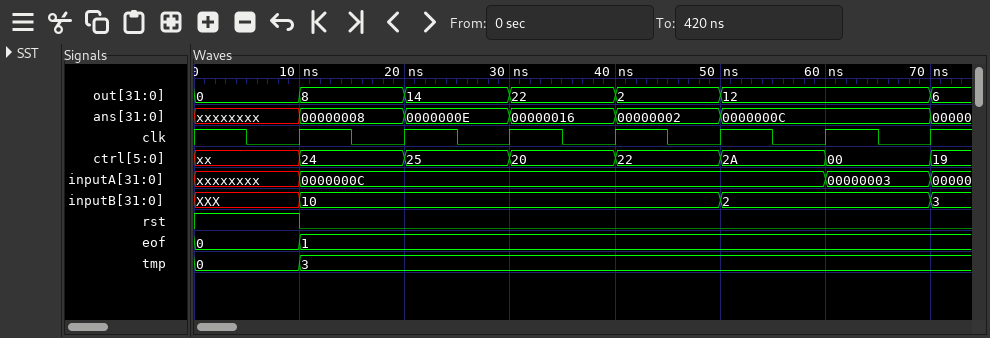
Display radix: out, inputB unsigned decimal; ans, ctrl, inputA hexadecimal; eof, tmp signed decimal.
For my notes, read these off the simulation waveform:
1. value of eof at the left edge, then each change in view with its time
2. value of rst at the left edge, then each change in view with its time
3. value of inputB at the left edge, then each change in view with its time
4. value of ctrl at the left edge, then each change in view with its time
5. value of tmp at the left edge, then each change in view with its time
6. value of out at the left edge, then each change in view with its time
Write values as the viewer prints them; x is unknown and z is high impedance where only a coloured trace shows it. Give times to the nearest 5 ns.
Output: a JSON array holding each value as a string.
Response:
["0, 1 at 10 ns", "1, 0 at 10 ns", "XXX, 10 at 10 ns, 2 at 50 ns, 3 at 70 ns", "xx, 24 at 10 ns, 25 at 20 ns, 20 at 30 ns, 22 at 40 ns, 2A at 50 ns, 00 at 60 ns, 19 at 70 ns", "0, 3 at 10 ns", "0, 8 at 10 ns, 14 at 20 ns, 22 at 30 ns, 2 at 40 ns, 12 at 50 ns, 6 at 70 ns"]
